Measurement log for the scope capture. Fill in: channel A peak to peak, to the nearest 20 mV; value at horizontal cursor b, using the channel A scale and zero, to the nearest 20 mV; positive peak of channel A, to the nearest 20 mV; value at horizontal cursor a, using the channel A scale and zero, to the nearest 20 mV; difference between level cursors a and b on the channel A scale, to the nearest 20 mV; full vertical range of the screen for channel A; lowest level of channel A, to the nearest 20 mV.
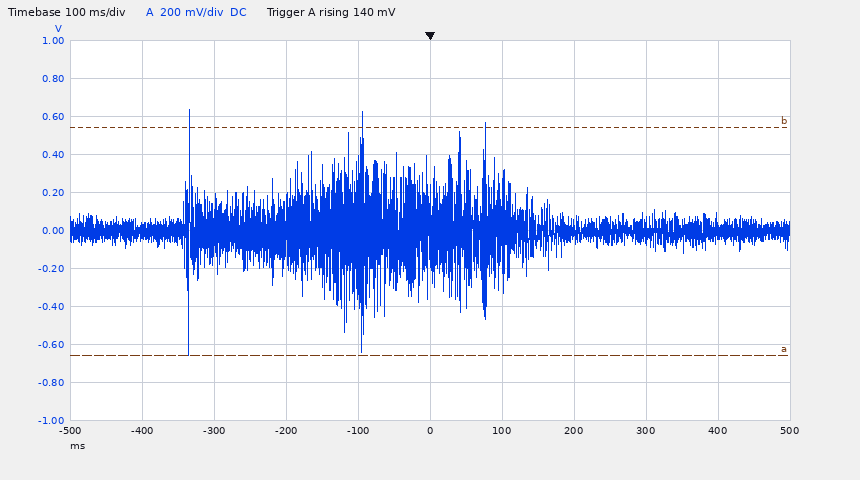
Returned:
1.30 V
540 mV
640 mV
-660 mV
1.20 V
2 V
-660 mV
